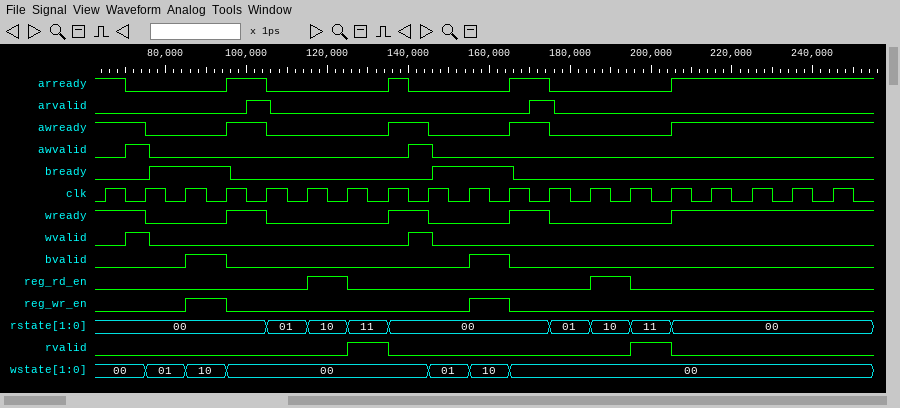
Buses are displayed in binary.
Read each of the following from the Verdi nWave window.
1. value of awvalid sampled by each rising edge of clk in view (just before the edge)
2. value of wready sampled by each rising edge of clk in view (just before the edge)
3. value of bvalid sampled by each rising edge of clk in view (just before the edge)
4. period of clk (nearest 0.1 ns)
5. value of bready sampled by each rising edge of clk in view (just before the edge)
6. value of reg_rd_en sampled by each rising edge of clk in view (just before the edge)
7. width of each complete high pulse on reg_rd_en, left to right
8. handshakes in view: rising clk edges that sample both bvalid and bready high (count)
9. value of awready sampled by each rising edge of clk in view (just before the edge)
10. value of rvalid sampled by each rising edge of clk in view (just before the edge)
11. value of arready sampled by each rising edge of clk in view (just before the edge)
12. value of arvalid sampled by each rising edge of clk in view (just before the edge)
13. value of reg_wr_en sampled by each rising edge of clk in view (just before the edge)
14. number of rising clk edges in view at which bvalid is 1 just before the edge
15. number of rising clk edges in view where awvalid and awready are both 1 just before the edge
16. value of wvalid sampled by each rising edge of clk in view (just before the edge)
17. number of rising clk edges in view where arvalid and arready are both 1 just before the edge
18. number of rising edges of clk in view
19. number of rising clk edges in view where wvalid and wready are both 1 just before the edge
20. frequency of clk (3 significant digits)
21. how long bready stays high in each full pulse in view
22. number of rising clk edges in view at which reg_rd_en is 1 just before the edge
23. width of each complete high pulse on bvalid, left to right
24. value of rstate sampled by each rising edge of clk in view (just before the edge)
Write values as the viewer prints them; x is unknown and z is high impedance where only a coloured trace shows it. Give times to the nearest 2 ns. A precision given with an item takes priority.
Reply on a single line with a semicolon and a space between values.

0 1 0 0 0 0 0 0 1 0 0 0 0 0 0 0 0 0 0; 1 1 0 0 1 0 0 0 1 0 0 1 0 0 0 1 1 1 1; 0 0 0 1 0 0 0 0 0 0 1 0 0 0 0 0 0 0 0; 10 ns; 0 0 1 1 0 0 0 0 0 1 1 0 0 0 0 0 0 0 0; 0 0 0 0 0 0 1 0 0 0 0 0 0 1 0 0 0 0 0; 10 ns, 10 ns; 2; 1 1 0 0 1 0 0 0 1 0 0 1 0 0 0 1 1 1 1; 0 0 0 0 0 0 0 1 0 0 0 0 0 0 1 0 0 0 0; 1 0 0 0 1 0 0 0 0 0 0 1 0 0 0 1 1 1 1; 0 0 0 0 1 0 0 0 0 0 0 1 0 0 0 0 0 0 0; 0 0 0 1 0 0 0 0 0 0 1 0 0 0 0 0 0 0 0; 2; 2; 0 1 0 0 0 0 0 0 1 0 0 0 0 0 0 0 0 0 0; 2; 19; 2; 100 MHz; 20 ns, 20 ns; 2; 10 ns, 10 ns; 00, 00, 00, 00, 00, 01, 10, 11, 00, 00, 00, 00, 01, 10, 11, 00, 00, 00, 00
